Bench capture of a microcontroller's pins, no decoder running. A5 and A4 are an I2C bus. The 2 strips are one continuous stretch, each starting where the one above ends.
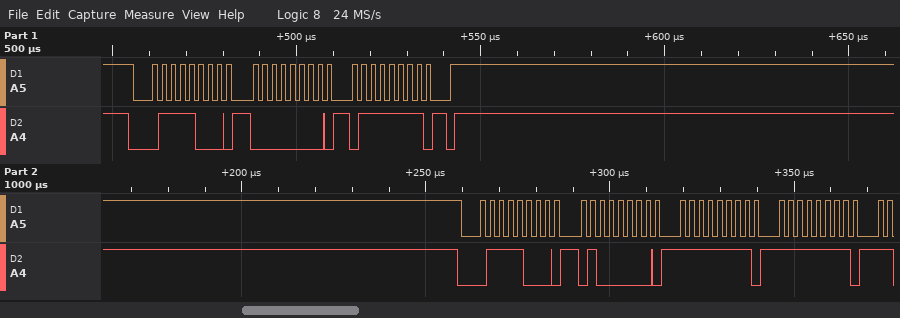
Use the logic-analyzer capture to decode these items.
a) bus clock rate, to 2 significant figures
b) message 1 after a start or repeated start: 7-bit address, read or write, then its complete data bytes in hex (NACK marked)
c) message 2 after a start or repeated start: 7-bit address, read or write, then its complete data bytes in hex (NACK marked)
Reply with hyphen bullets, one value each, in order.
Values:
- 400 kHz
- 0x3C write: 00 7F
- 0x3C write: 40 FF FF
